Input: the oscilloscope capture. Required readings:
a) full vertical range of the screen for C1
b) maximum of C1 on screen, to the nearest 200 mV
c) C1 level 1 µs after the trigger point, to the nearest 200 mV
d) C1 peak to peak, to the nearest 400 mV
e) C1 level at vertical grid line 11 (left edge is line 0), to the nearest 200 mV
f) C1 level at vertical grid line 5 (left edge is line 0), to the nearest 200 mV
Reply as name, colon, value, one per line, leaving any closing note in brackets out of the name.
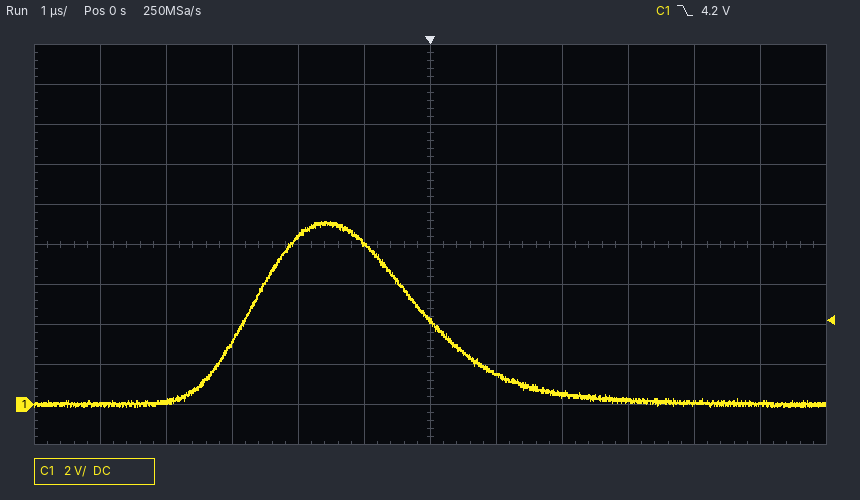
full vertical range of the screen for C1: 20 V
maximum of C1 on screen, to the nearest 200 mV: 9.2 V
C1 level 1 µs after the trigger point, to the nearest 200 mV: 1.6 V
C1 peak to peak, to the nearest 400 mV: 9.2 V
C1 level at vertical grid line 11 (left edge is line 0), to the nearest 200 mV: 0.0 V
C1 level at vertical grid line 5 (left edge is line 0), to the nearest 200 mV: 8.0 V
